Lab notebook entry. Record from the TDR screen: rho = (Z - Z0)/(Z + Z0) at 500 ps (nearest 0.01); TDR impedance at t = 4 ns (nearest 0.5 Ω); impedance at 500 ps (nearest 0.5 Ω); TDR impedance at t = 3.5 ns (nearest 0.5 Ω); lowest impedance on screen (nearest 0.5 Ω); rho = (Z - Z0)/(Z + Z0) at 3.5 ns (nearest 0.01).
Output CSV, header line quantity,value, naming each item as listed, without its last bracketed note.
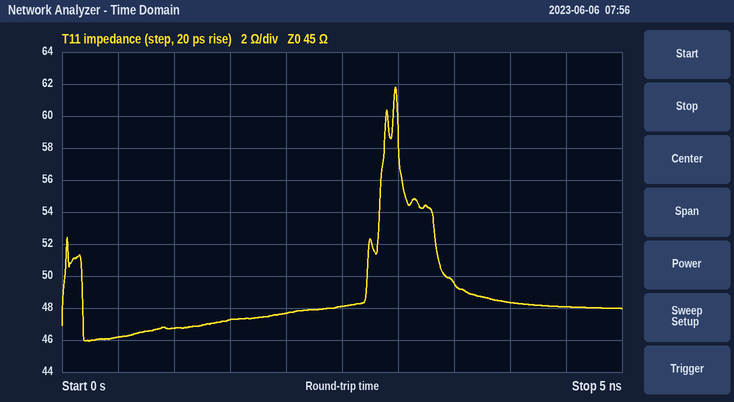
quantity,value
rho = (Z - Z0)/(Z + Z0) at 500 ps,+0.01
TDR impedance at t = 4 ns,48.5 Ω
impedance at 500 ps,46.0 Ω
TDR impedance at t = 3.5 ns,49.5 Ω
lowest impedance on screen,46.0 Ω
rho = (Z - Z0)/(Z + Z0) at 3.5 ns,+0.05
